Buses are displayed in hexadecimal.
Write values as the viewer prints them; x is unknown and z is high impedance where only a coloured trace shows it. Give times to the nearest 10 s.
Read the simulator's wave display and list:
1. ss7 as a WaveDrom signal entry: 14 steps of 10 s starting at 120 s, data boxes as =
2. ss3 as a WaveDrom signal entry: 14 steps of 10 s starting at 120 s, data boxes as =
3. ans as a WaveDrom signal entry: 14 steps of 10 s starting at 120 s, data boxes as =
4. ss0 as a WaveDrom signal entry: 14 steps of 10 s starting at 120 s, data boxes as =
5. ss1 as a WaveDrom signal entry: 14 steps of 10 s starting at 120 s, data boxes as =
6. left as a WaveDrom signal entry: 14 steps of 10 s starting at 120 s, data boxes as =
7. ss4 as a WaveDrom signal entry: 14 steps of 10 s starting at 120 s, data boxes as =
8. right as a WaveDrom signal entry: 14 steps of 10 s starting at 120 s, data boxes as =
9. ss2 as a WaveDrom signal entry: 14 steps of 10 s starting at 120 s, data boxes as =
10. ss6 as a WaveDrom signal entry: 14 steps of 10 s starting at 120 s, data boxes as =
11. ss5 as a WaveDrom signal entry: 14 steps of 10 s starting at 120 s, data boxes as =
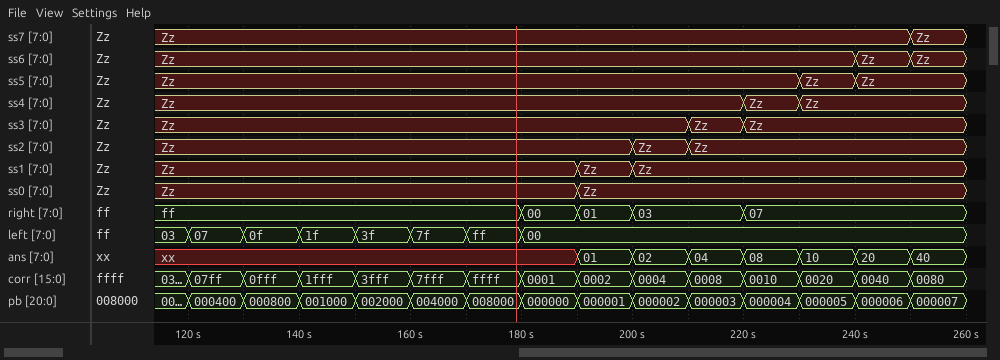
{name: 'ss7', wave: '=............=', data: 'Zz Zz'}
{name: 'ss3', wave: '=........==...', data: 'Zz Zz Zz'}
{name: 'ans', wave: 'x......=======', data: '01 02 04 08 10 20 40'}
{name: 'ss0', wave: '=......=......', data: 'Zz Zz'}
{name: 'ss1', wave: '=......==.....', data: 'Zz Zz Zz'}
{name: 'left', wave: '=======.......', data: '07 0f 1f 3f 7f ff 00'}
{name: 'ss4', wave: '=.........==..', data: 'Zz Zz Zz'}
{name: 'right', wave: '=.....===.=...', data: 'ff 00 01 03 07'}
{name: 'ss2', wave: '=.......==....', data: 'Zz Zz Zz'}
{name: 'ss6', wave: '=...........==', data: 'Zz Zz Zz'}
{name: 'ss5', wave: '=..........==.', data: 'Zz Zz Zz'}
